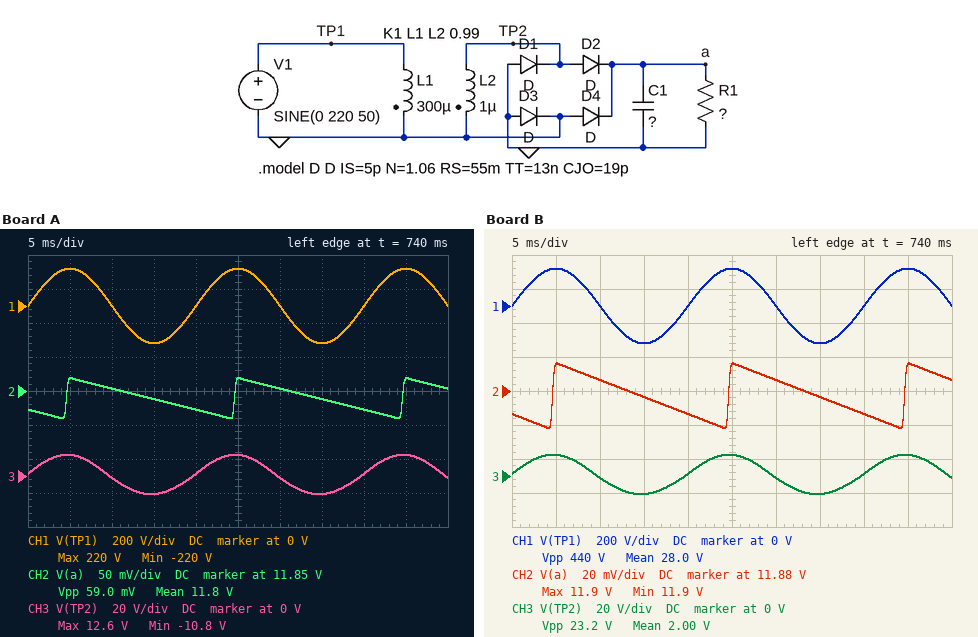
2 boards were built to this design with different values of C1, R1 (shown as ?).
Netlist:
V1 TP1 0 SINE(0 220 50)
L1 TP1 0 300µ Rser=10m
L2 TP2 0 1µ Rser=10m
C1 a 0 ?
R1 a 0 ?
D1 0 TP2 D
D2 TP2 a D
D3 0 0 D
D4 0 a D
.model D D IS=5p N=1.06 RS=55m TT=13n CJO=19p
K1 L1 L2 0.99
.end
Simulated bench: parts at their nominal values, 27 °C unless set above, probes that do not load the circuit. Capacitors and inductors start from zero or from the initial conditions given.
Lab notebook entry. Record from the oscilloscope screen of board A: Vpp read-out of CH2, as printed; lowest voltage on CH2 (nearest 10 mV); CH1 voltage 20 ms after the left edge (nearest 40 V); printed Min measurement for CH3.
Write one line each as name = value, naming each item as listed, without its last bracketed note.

Vpp read-out of CH2, as printed = 59.0 mV
lowest voltage on CH2 = 11.81 V
CH1 voltage 20 ms after the left edge = 0 V
printed Min measurement for CH3 = -10.8 V
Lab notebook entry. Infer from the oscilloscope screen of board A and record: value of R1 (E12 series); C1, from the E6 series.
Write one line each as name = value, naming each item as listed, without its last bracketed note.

value of R1 = 5.6 kΩ
C1, from the E6 series = 680 µF
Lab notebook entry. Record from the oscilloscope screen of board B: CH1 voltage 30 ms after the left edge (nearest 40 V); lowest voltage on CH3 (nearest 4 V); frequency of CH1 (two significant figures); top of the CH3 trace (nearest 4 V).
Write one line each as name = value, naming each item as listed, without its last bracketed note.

CH1 voltage 30 ms after the left edge = 0 V
lowest voltage on CH3 = -12 V
frequency of CH1 = 50 Hz
top of the CH3 trace = 12 V
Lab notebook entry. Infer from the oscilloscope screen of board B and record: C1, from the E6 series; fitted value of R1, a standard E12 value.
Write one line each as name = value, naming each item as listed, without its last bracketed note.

C1, from the E6 series = 330 µF
fitted value of R1, a standard E12 value = 18 kΩ
